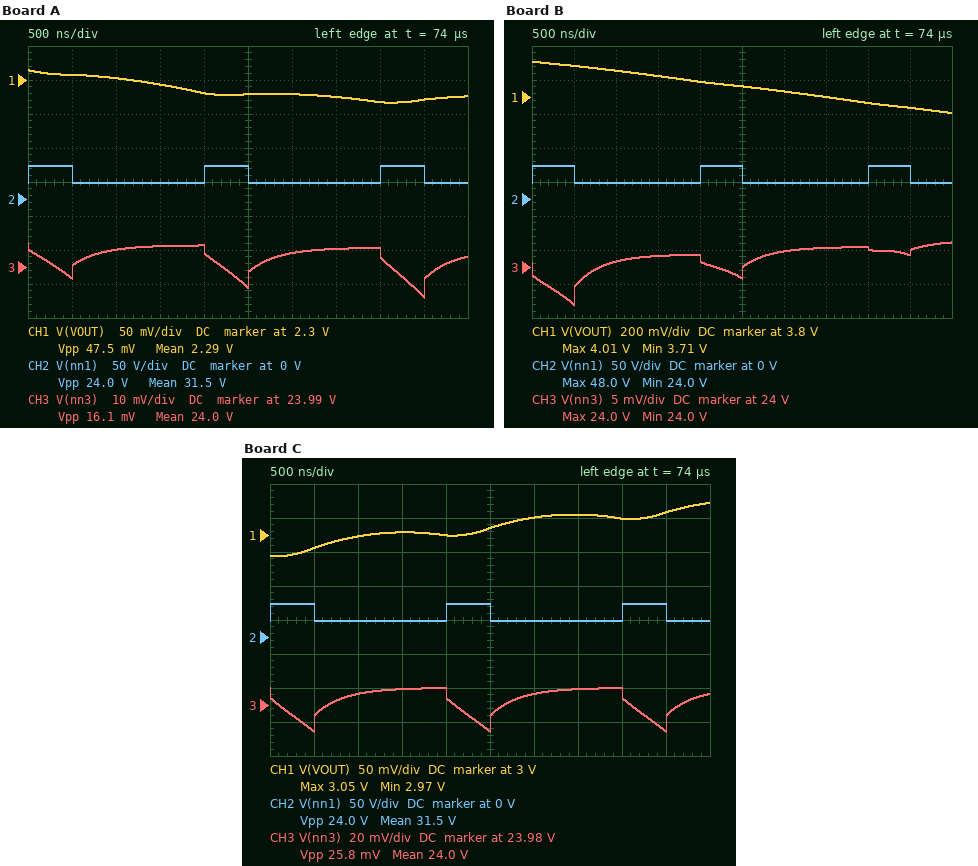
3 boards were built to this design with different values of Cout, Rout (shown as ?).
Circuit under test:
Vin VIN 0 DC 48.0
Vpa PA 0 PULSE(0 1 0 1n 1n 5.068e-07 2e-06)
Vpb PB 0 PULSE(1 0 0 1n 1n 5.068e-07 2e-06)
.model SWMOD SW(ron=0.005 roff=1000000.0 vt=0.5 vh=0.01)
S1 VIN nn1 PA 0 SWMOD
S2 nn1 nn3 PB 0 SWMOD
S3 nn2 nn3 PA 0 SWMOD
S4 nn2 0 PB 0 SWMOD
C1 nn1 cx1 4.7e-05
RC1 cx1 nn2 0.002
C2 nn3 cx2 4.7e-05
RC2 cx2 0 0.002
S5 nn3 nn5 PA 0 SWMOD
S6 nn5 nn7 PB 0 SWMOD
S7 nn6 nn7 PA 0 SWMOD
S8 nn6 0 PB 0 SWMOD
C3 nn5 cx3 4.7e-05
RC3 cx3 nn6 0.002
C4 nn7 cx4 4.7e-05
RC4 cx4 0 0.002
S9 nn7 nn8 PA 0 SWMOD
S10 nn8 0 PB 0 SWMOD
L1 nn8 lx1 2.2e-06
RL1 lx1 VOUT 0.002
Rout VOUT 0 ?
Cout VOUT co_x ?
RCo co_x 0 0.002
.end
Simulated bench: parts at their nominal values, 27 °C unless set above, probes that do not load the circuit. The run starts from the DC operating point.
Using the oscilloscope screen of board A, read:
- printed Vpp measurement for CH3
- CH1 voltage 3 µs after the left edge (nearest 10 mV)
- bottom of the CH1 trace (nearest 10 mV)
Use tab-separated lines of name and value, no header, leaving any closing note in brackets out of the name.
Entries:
printed Vpp measurement for CH3	16.1 mV
CH1 voltage 3 µs after the left edge	2.28 V
bottom of the CH1 trace	2.27 V
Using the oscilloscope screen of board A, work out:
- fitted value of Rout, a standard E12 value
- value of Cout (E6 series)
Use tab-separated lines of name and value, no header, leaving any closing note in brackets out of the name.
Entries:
fitted value of Rout, a standard E12 value	0.47 Ω
value of Cout	68 µF
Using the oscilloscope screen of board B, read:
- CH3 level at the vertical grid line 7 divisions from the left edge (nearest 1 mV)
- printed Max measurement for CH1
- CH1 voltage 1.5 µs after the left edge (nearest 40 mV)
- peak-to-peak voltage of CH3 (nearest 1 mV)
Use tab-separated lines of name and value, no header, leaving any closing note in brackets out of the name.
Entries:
CH3 level at the vertical grid line 7 divisions from the left edge	23.998 V
printed Max measurement for CH1	4.01 V
CH1 voltage 1.5 µs after the left edge	3.92 V
peak-to-peak voltage of CH3	9 mV
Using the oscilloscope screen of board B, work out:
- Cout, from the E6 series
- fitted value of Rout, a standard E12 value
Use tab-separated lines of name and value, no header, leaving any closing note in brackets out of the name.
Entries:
Cout, from the E6 series	150 µF
fitted value of Rout, a standard E12 value	0.39 Ω
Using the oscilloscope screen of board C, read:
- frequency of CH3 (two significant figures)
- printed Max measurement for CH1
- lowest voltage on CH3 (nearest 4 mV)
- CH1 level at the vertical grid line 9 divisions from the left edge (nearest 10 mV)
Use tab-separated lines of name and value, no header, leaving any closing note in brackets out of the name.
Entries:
frequency of CH3	500 kHz
printed Max measurement for CH1	3.05 V
lowest voltage on CH3	23.964 V
CH1 level at the vertical grid line 9 divisions from the left edge	3.03 V
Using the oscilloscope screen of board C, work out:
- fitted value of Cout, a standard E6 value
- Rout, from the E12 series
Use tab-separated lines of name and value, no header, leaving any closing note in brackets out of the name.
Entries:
fitted value of Cout, a standard E6 value	33 µF
Rout, from the E12 series	0.39 Ω
